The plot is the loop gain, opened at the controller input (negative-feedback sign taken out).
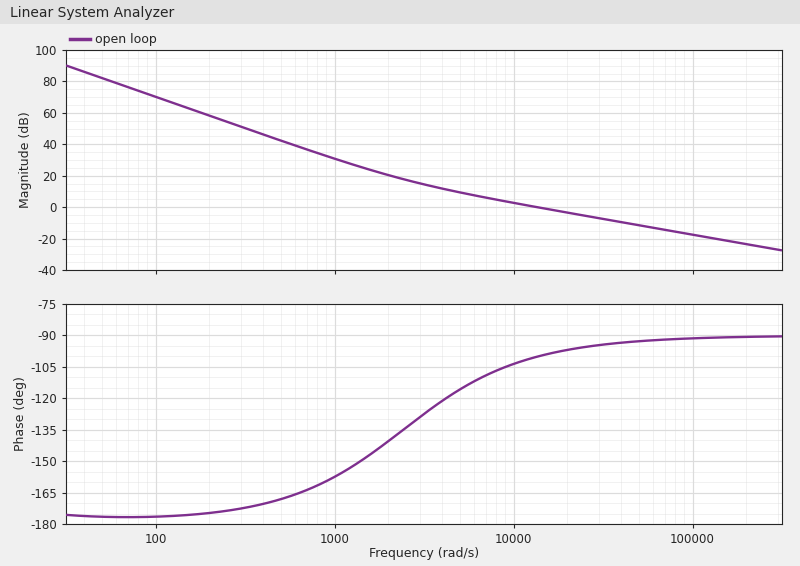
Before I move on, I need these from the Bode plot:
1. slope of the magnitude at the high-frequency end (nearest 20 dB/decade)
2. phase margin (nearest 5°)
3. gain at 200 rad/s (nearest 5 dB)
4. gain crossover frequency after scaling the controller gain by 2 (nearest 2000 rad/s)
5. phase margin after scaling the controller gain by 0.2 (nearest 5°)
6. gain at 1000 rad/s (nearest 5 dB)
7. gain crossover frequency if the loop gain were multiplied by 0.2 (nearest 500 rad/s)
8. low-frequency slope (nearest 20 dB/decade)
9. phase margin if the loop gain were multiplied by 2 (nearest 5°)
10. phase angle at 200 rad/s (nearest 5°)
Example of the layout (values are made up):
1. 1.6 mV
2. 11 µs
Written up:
1. -20 dB/decade
2. 80°
3. 60 dB
4. 26000 rad/s
5. 55°
6. 30 dB
7. 3500 rad/s
8. -40 dB/decade
9. 85°
10. -175°
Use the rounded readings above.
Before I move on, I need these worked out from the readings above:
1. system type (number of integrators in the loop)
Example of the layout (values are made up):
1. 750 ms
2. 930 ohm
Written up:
1. 2
